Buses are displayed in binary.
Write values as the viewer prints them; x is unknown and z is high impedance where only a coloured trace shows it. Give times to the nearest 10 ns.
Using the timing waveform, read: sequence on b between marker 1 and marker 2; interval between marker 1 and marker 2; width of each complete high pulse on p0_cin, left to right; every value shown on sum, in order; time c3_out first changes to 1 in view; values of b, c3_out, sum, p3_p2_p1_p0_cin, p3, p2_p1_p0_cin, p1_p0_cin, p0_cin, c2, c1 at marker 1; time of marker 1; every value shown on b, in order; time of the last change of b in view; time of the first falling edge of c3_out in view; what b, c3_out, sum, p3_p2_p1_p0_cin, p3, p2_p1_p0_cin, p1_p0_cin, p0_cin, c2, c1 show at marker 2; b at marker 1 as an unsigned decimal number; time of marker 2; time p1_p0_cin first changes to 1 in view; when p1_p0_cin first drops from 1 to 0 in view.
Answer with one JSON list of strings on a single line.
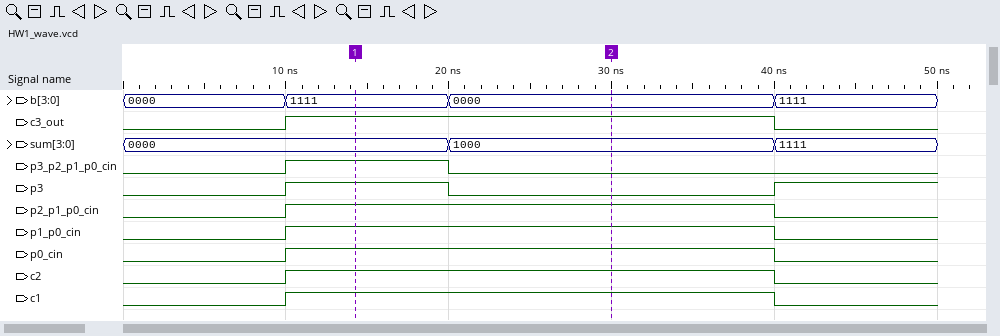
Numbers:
["1111, 0000", "20 ns", "30 ns", "0000, 1000, 1111", "10 ns", "b=1111, c3_out=1, sum=0000, p3_p2_p1_p0_cin=1, p3=1, p2_p1_p0_cin=1, p1_p0_cin=1, p0_cin=1, c2=1, c1=1", "10 ns", "0000, 1111, 0000, 1111", "40 ns", "40 ns", "b=0000, c3_out=1, sum=1000, p3_p2_p1_p0_cin=0, p3=0, p2_p1_p0_cin=1, p1_p0_cin=1, p0_cin=1, c2=1, c1=1", "15", "30 ns", "10 ns", "40 ns"]
